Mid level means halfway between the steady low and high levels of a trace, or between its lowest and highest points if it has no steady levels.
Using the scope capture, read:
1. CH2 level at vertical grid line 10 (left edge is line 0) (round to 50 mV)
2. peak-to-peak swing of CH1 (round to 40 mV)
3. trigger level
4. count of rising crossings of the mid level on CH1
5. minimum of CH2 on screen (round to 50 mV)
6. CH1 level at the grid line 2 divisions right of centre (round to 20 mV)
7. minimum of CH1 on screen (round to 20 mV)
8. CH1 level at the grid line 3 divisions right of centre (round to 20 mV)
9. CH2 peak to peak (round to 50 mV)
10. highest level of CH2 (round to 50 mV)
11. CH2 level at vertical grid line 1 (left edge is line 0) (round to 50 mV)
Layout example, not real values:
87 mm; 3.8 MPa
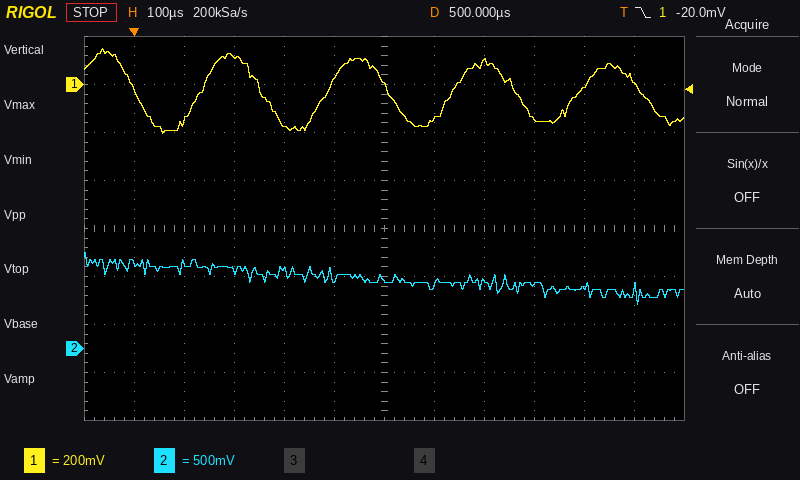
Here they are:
650 mV; 360 mV; -20.0 mV; 4; 450 mV; 100 mV; -200 mV; -140 mV; 550 mV; 1.00 V; 900 mV
